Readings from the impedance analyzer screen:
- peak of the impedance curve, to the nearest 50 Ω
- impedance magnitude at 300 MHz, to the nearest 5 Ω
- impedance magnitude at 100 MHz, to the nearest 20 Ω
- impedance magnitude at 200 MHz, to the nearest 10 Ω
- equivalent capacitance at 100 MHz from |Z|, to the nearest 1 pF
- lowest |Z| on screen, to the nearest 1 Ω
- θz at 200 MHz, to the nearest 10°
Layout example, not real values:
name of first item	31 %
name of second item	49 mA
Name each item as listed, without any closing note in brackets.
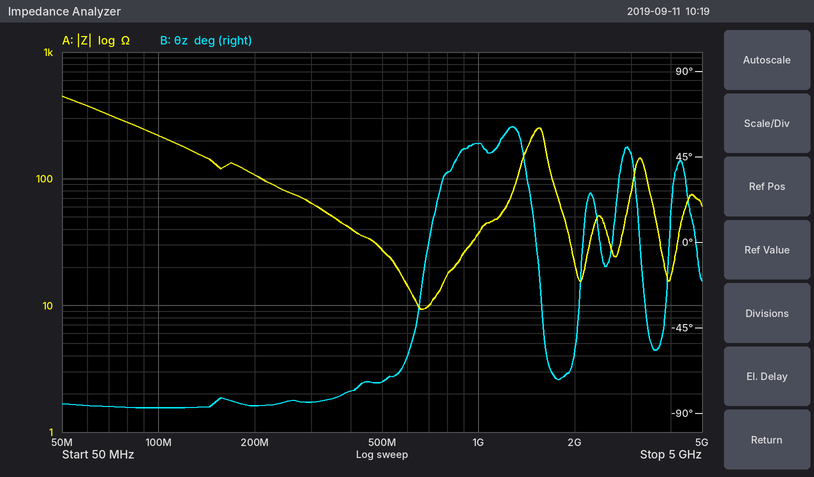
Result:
peak of the impedance curve, to the nearest 50 Ω	450 Ω
impedance magnitude at 300 MHz, to the nearest 5 Ω	65 Ω
impedance magnitude at 100 MHz, to the nearest 20 Ω	220 Ω
impedance magnitude at 200 MHz, to the nearest 10 Ω	110 Ω
equivalent capacitance at 100 MHz from |Z|, to the nearest 1 pF	7 pF
lowest |Z| on screen, to the nearest 1 Ω	9 Ω
θz at 200 MHz, to the nearest 10°	-90°
